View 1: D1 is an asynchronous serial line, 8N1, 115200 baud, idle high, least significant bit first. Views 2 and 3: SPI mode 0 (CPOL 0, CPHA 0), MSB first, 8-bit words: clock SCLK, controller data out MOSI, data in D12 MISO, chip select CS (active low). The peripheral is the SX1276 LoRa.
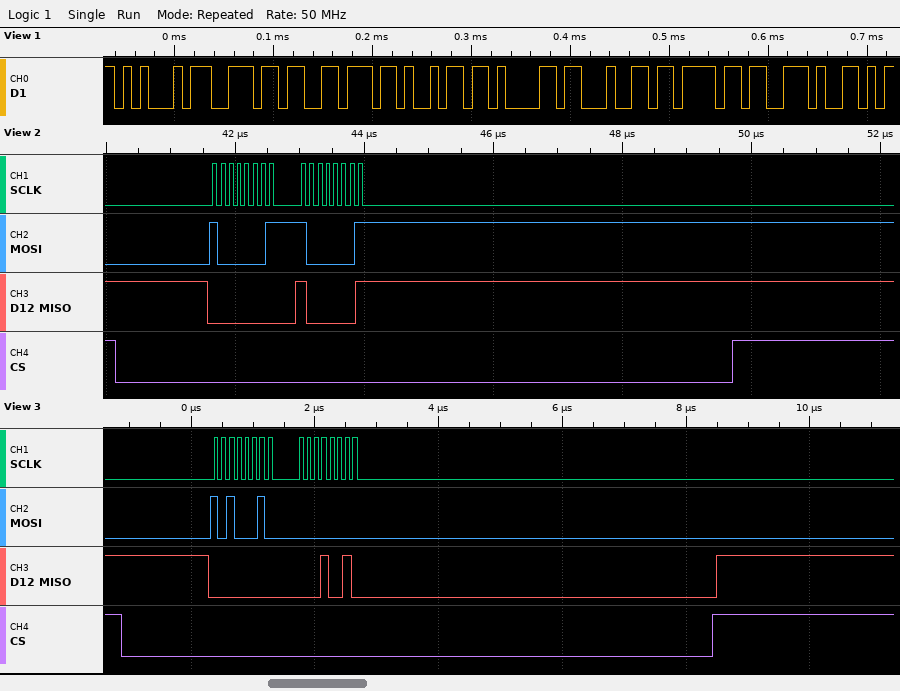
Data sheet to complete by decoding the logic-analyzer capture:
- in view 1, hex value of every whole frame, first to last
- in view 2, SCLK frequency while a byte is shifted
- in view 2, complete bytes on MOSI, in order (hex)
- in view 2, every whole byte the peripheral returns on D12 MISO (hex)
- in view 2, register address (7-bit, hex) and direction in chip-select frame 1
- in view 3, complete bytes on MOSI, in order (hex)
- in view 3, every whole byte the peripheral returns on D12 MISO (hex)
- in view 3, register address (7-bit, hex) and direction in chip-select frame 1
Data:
45 6E 76 69 61 64 6F 2E
8 MHz
0x81 0x81
0x00 0x81
0x01 write
A2 00
00 12
0x22 write
